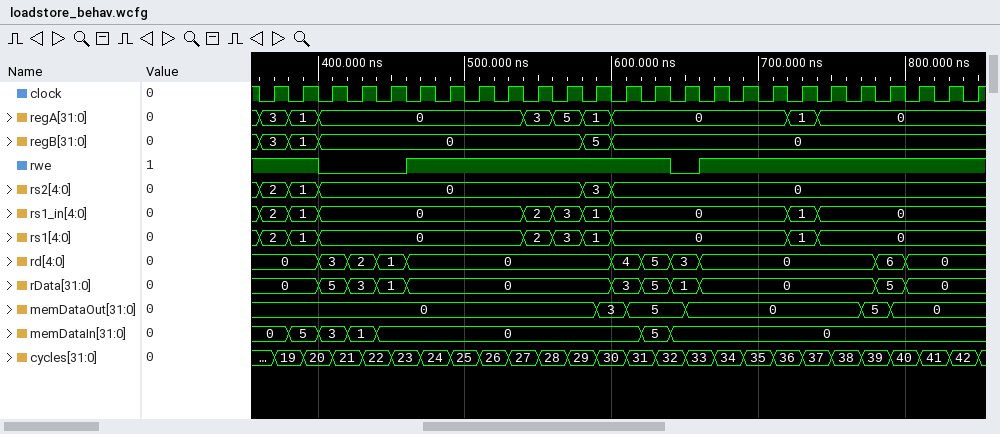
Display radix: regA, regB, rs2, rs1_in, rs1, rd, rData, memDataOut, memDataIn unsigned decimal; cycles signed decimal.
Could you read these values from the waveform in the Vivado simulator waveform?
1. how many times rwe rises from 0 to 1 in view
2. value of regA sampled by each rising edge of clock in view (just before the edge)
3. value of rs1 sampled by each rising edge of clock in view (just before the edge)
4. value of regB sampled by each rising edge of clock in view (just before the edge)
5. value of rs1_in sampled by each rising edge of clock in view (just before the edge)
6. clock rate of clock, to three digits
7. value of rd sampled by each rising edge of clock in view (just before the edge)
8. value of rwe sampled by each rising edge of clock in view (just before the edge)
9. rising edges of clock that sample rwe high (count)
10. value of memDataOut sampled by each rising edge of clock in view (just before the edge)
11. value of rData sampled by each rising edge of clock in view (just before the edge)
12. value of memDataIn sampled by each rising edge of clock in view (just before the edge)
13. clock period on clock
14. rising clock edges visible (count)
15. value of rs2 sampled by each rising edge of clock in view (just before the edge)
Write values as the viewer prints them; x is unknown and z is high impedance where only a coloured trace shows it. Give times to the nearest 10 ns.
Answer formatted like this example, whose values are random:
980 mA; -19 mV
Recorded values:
2; 3, 1, 0, 0, 0, 0, 0, 0, 0, 3, 5, 1, 0, 0, 0, 0, 0, 0, 1, 0, 0, 0, 0, 0, 0; 2, 1, 0, 0, 0, 0, 0, 0, 0, 2, 3, 1, 0, 0, 0, 0, 0, 0, 1, 0, 0, 0, 0, 0, 0; 3, 1, 0, 0, 0, 0, 0, 0, 0, 0, 0, 5, 0, 0, 0, 0, 0, 0, 0, 0, 0, 0, 0, 0, 0; 2, 1, 0, 0, 0, 0, 0, 0, 0, 2, 3, 1, 0, 0, 0, 0, 0, 0, 1, 0, 0, 0, 0, 0, 0; 50.0 MHz; 0, 0, 3, 2, 1, 0, 0, 0, 0, 0, 0, 0, 4, 5, 3, 0, 0, 0, 0, 0, 0, 6, 0, 0, 0; 1 1 0 0 0 1 1 1 1 1 1 1 1 1 0 1 1 1 1 1 1 1 1 1 1; 21; 0, 0, 0, 0, 0, 0, 0, 0, 0, 0, 0, 0, 3, 5, 5, 0, 0, 0, 0, 0, 0, 5, 0, 0, 0; 0, 0, 5, 3, 1, 0, 0, 0, 0, 0, 0, 0, 3, 5, 1, 0, 0, 0, 0, 0, 0, 5, 0, 0, 0; 0, 5, 3, 1, 0, 0, 0, 0, 0, 0, 0, 0, 0, 5, 0, 0, 0, 0, 0, 0, 0, 0, 0, 0, 0; 20 ns; 25; 2, 1, 0, 0, 0, 0, 0, 0, 0, 0, 0, 3, 0, 0, 0, 0, 0, 0, 0, 0, 0, 0, 0, 0, 0
